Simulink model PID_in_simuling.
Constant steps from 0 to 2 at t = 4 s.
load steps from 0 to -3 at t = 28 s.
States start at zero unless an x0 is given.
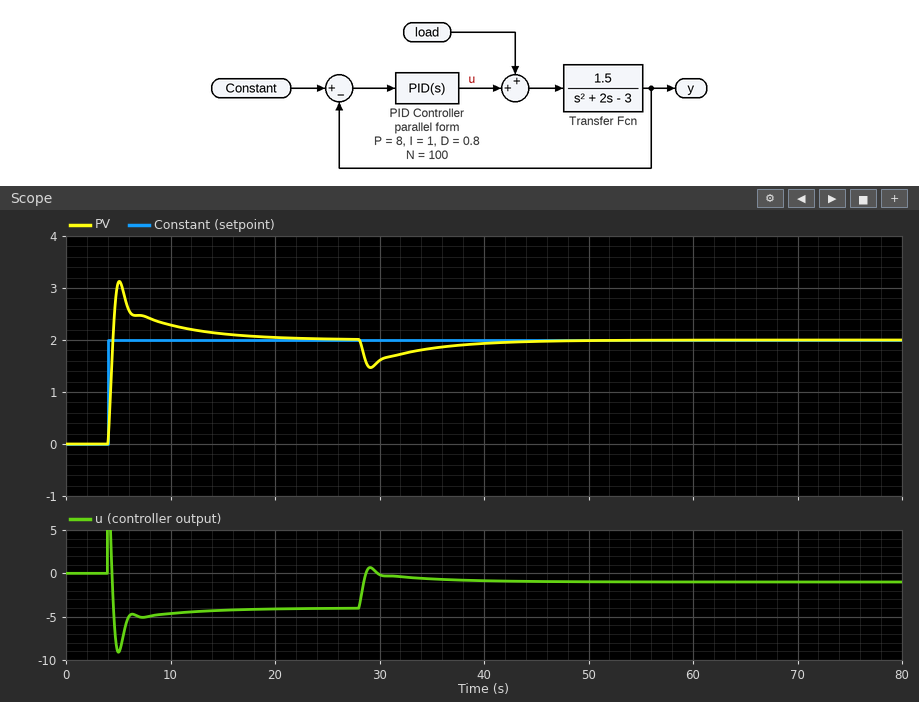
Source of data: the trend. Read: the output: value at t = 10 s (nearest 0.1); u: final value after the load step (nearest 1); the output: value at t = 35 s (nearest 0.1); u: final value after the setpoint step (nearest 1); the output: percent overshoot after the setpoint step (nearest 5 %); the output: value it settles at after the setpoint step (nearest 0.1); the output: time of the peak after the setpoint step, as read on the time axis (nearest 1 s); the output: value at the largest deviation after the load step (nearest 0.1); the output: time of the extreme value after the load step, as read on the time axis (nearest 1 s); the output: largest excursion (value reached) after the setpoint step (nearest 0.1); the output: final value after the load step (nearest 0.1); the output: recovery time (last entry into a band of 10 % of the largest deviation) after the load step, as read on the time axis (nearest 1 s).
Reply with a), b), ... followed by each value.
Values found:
a) 2.3
b) -1
c) 1.8
d) -4
e) 55 %
f) 2.0
g) 5 s
h) 1.5
i) 29 s
j) 3.1
k) 2.0
l) 41 s
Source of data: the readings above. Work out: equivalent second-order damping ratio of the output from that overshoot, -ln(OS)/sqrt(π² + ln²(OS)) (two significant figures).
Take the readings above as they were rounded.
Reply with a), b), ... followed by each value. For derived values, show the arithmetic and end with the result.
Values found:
a) ln(0.55) = -0.598; 0.598 / sqrt(9.870 + 0.357) = 0.19
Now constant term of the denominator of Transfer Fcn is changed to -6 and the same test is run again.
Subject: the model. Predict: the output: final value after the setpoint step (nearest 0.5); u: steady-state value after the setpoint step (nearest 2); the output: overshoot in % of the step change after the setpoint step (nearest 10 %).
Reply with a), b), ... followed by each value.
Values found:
a) 2.0
b) -8
c) 110 %
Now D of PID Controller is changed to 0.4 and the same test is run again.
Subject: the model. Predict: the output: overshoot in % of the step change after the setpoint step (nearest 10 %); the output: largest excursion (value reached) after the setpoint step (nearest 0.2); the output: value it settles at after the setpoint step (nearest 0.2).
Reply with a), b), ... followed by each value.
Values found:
a) 70 %
b) 3.4
c) 2.0
